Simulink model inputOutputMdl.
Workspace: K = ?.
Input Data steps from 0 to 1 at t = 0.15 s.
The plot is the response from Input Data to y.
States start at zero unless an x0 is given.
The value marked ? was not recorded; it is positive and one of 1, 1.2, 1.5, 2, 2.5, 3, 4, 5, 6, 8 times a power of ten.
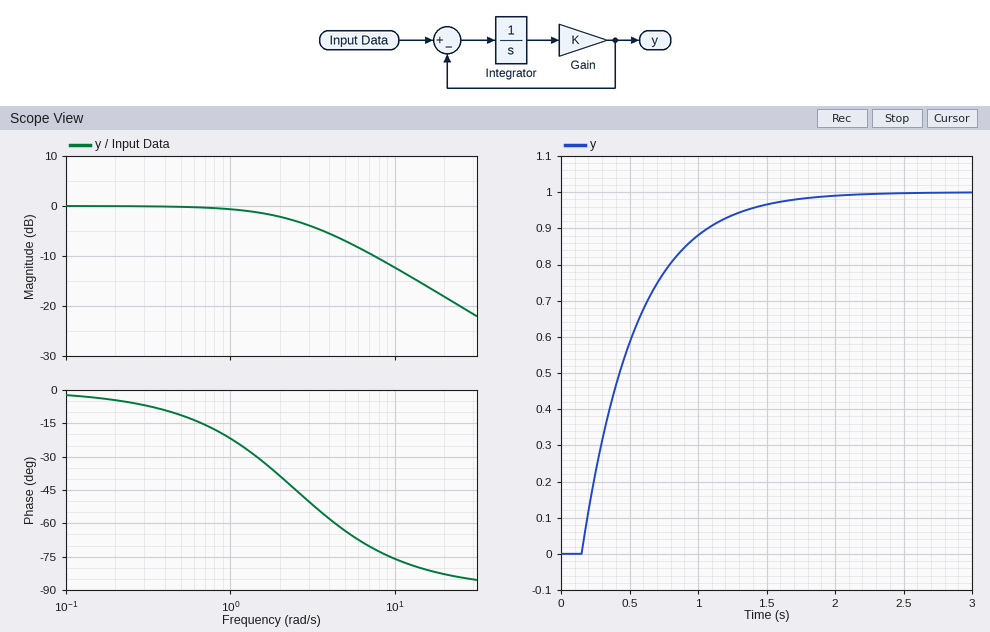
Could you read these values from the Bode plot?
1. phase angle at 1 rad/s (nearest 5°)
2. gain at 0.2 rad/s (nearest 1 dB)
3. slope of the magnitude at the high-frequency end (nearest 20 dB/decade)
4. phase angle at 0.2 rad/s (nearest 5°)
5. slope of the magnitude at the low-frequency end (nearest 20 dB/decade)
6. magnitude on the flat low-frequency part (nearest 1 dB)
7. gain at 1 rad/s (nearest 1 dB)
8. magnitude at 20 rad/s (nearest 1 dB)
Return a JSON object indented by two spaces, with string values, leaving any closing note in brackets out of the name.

{
  "phase angle at 1 rad/s": "-20°",
  "gain at 0.2 rad/s": "0 dB",
  "slope of the magnitude at the high-frequency end": "-20 dB/decade",
  "phase angle at 0.2 rad/s": "-5°",
  "slope of the magnitude at the low-frequency end": "0 dB/decade",
  "magnitude on the flat low-frequency part": "0 dB",
  "gain at 1 rad/s": "-1 dB",
  "magnitude at 20 rad/s": "-18 dB"
}
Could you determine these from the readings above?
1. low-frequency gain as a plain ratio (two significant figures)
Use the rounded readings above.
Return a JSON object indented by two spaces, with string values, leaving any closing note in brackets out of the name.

{
  "low-frequency gain as a plain ratio": "1.0"
}
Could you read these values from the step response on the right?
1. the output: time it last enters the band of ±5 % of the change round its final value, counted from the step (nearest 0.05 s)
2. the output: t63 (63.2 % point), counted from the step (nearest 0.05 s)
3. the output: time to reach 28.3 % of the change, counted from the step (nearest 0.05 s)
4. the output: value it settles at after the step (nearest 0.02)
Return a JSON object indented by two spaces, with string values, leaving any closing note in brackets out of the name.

{
  "the output: time it last enters the band of ±5 % of the change round its final value, counted from the step": "1.20 s",
  "the output: t63 (63.2 % point), counted from the step": "0.40 s",
  "the output: time to reach 28.3 % of the change, counted from the step": "0.15 s",
  "the output: value it settles at after the step": "1.00"
}
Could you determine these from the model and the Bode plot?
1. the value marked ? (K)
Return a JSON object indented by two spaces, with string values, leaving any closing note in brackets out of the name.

{
  "the value marked ?": "2.5"
}
